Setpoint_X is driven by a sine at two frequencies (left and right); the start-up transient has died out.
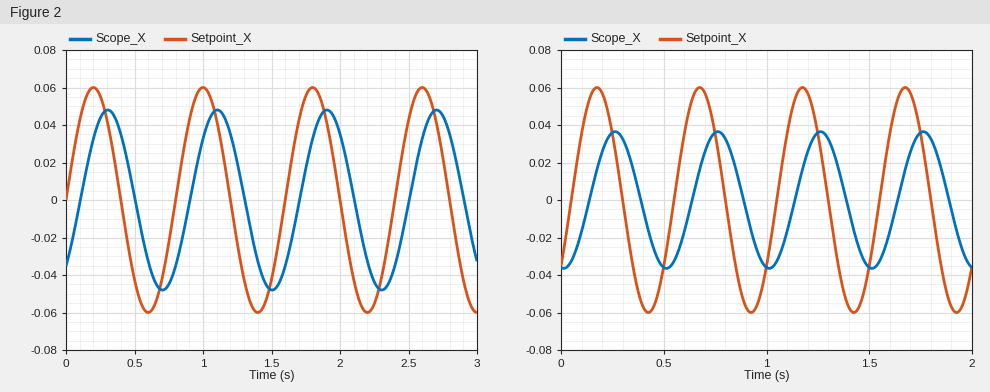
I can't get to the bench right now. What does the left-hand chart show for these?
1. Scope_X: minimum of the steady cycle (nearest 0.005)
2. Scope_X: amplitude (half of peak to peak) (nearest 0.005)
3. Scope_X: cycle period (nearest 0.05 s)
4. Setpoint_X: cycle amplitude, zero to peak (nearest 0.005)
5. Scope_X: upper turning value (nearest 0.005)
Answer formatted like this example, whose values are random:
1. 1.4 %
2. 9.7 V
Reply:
1. -0.050
2. 0.050
3. 0.80 s
4. 0.060
5. 0.050
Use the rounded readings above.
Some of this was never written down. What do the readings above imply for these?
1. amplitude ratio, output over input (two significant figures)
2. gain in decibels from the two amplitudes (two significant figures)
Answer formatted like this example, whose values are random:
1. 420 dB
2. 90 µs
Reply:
1. 0.83
2. -1.6 dB
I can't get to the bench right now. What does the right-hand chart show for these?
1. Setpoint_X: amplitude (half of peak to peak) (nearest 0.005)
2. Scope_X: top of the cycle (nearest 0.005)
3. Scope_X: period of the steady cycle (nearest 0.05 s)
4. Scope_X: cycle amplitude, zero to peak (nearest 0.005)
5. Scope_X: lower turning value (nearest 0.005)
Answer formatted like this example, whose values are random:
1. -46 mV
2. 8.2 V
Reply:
1. 0.060
2. 0.035
3. 0.50 s
4. 0.035
5. -0.035
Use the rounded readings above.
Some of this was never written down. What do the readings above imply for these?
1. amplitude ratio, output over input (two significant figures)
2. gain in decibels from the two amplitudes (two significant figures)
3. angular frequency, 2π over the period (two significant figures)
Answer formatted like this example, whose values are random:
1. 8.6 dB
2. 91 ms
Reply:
1. 0.58
2. -4.7 dB
3. 13 rad/s
